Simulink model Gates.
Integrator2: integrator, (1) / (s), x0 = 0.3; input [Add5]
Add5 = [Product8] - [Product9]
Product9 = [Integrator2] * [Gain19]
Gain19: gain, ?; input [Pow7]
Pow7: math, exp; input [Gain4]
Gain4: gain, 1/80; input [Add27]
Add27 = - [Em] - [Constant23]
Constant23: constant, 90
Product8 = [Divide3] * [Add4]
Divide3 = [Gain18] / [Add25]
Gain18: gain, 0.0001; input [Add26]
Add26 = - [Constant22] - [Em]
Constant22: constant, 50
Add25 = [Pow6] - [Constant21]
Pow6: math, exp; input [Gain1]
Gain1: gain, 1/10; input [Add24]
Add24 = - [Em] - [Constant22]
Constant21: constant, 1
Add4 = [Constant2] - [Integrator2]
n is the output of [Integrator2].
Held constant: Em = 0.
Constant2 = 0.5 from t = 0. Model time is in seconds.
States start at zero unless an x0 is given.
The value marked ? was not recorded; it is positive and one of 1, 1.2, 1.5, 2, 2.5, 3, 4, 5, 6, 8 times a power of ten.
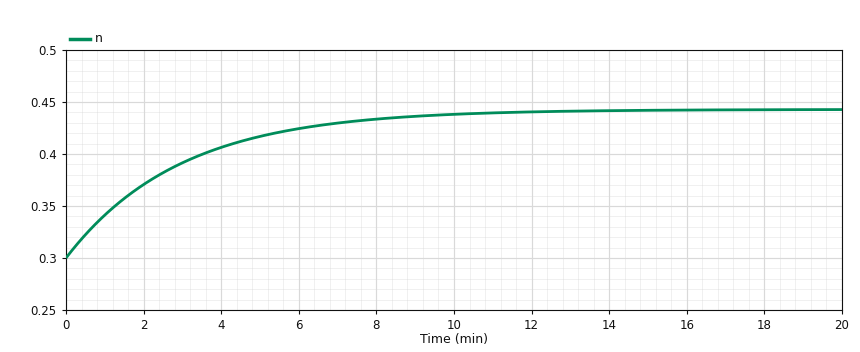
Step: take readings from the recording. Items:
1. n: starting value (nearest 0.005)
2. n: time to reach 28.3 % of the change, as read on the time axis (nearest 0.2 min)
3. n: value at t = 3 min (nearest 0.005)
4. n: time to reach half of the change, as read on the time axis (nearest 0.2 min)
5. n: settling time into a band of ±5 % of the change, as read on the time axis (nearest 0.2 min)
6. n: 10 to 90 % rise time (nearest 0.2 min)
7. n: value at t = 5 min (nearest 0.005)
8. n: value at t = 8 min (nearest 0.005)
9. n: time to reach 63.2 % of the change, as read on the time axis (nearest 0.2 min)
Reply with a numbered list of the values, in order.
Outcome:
1. 0.300
2. 1.0 min
3. 0.390
4. 2.0 min
5. 8.8 min
6. 6.4 min
7. 0.415
8. 0.435
9. 3.0 min
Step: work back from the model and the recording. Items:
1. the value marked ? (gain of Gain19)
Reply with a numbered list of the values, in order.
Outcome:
1. 0.002
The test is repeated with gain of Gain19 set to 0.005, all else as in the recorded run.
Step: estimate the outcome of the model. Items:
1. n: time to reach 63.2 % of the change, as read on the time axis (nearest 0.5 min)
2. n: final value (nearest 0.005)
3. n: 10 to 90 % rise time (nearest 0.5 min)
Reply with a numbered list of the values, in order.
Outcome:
1. 2.5 min
2. 0.380
3. 5.5 min
